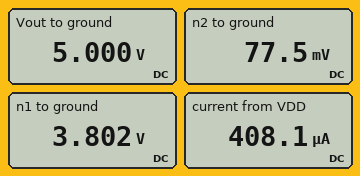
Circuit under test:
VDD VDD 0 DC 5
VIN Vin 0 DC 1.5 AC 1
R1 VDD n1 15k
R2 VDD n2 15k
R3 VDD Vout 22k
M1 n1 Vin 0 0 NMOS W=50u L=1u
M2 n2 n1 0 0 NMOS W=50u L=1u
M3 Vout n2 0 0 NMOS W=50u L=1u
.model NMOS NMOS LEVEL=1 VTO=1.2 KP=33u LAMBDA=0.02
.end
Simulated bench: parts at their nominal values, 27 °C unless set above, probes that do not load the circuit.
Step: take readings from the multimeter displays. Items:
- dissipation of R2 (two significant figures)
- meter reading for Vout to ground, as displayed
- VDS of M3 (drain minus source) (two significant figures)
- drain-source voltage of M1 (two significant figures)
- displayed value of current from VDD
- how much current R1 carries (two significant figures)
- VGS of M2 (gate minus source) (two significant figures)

1.6 mW
5.000 V
5.0 V
3.8 V
408.1 µA
80 µA
3.8 V
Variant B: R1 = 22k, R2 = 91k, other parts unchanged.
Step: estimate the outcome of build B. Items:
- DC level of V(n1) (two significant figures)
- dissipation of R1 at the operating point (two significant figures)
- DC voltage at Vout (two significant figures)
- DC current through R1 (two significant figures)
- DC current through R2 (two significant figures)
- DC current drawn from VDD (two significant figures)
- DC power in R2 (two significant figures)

3.3 V
140 µW
5.0 V
79 µA
55 µA
130 µA
270 µW
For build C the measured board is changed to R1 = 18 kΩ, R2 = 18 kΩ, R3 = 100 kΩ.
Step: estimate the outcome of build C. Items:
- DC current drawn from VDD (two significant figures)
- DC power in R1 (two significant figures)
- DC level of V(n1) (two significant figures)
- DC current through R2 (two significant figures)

350 µA
110 µW
3.6 V
270 µA
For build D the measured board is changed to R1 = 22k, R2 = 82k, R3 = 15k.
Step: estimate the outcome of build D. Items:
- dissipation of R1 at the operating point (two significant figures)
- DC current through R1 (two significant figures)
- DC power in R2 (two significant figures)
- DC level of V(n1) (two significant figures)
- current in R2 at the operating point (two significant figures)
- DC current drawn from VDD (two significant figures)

140 µW
79 µA
300 µW
3.3 V
61 µA
140 µA
